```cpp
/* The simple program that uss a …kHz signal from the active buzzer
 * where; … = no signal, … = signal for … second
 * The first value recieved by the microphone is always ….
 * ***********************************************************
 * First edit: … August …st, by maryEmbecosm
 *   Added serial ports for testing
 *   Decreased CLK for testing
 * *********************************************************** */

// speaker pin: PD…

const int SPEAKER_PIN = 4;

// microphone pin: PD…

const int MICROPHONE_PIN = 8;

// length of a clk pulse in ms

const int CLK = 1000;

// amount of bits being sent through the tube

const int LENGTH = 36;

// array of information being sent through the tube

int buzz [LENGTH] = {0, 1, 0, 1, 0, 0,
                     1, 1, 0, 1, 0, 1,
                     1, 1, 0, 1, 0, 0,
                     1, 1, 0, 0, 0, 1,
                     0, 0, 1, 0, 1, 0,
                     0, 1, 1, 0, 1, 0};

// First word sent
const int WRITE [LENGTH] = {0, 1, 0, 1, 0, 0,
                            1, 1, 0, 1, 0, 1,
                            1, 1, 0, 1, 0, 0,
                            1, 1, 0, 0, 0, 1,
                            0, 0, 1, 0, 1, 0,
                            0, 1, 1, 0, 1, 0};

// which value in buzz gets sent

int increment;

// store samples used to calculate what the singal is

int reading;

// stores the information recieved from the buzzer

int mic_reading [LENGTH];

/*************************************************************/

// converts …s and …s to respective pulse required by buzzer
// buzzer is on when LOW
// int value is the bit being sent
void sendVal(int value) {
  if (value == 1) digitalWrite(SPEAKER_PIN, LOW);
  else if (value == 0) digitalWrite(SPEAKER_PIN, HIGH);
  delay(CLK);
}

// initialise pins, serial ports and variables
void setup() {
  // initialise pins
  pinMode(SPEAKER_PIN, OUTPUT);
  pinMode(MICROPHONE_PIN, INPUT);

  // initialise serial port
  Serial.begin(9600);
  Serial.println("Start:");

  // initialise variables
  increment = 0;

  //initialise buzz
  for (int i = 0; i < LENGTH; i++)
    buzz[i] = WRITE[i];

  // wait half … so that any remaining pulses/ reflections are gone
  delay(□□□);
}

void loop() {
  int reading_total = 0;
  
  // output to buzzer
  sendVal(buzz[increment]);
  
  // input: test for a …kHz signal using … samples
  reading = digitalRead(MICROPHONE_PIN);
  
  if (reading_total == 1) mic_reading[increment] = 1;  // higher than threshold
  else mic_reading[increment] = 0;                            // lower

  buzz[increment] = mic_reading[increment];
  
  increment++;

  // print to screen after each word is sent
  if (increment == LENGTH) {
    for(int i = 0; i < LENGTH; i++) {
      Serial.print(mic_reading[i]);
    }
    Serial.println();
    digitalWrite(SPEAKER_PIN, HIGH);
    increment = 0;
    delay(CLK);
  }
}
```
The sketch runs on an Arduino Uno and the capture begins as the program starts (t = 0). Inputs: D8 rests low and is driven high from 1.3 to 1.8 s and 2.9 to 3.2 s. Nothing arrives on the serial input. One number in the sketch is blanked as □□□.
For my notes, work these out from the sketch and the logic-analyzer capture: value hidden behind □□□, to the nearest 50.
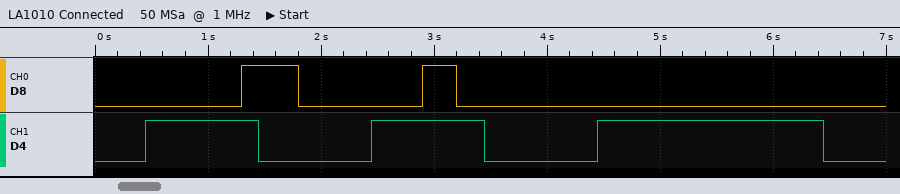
450
